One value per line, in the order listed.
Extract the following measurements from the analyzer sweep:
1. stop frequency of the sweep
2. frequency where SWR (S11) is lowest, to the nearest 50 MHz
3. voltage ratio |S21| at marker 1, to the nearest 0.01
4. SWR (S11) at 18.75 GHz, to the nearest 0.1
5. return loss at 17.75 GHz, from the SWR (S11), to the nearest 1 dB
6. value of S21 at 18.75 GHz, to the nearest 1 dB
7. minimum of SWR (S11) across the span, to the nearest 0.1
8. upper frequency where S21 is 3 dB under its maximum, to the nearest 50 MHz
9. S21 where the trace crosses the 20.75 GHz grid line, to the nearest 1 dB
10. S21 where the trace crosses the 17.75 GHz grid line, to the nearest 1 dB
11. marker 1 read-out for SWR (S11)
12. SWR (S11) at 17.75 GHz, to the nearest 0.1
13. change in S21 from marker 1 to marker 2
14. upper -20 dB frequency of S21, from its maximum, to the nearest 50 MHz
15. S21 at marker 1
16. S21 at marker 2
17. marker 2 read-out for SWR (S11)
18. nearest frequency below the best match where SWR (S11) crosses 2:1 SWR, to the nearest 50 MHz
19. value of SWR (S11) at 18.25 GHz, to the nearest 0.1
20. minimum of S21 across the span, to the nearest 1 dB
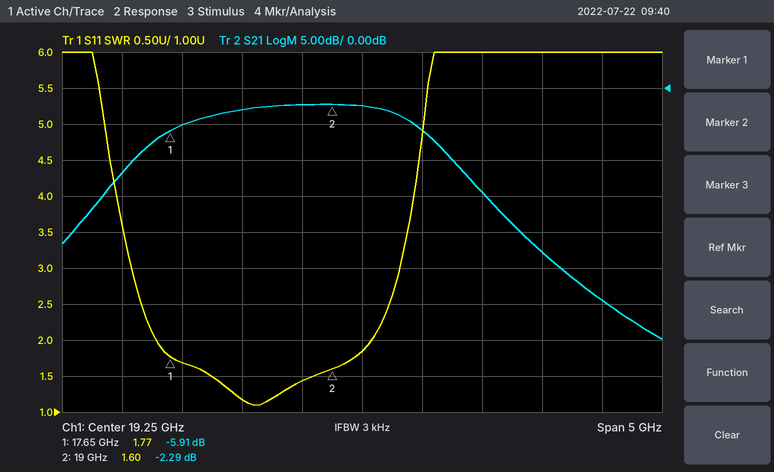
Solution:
21.75 GHz
18.35 GHz
0.51
1.4
12 dB
-2 dB
1.1
19.70 GHz
-23 dB
-5 dB
1.77
1.7
3.62 dB
20.70 GHz
-5.91 dB
-2.29 dB
1.60
17.55 GHz
1.2
-35 dB
